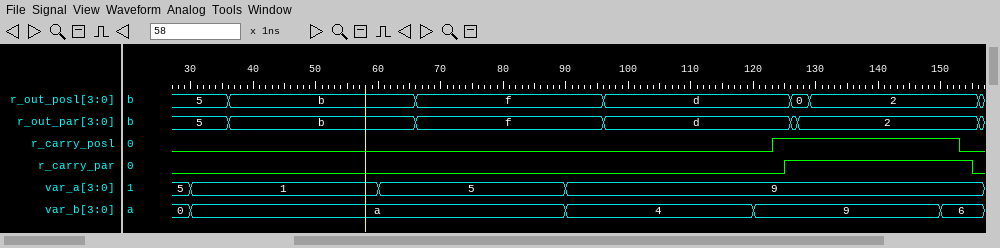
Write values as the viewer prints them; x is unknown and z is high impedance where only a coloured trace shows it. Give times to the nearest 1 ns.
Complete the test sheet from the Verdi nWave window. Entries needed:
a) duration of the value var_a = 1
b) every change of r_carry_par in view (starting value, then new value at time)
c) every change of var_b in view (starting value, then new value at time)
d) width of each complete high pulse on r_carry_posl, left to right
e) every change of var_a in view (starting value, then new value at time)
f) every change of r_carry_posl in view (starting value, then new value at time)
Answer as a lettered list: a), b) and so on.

a) 30 ns
b) 0, 1 at 125 ns, 0 at 155 ns
c) 0, a at 30 ns, 4 at 90 ns, 9 at 120 ns, 6 at 150 ns
d) 30 ns
e) 5, 1 at 30 ns, 5 at 60 ns, 9 at 90 ns
f) 0, 1 at 123 ns, 0 at 153 ns
